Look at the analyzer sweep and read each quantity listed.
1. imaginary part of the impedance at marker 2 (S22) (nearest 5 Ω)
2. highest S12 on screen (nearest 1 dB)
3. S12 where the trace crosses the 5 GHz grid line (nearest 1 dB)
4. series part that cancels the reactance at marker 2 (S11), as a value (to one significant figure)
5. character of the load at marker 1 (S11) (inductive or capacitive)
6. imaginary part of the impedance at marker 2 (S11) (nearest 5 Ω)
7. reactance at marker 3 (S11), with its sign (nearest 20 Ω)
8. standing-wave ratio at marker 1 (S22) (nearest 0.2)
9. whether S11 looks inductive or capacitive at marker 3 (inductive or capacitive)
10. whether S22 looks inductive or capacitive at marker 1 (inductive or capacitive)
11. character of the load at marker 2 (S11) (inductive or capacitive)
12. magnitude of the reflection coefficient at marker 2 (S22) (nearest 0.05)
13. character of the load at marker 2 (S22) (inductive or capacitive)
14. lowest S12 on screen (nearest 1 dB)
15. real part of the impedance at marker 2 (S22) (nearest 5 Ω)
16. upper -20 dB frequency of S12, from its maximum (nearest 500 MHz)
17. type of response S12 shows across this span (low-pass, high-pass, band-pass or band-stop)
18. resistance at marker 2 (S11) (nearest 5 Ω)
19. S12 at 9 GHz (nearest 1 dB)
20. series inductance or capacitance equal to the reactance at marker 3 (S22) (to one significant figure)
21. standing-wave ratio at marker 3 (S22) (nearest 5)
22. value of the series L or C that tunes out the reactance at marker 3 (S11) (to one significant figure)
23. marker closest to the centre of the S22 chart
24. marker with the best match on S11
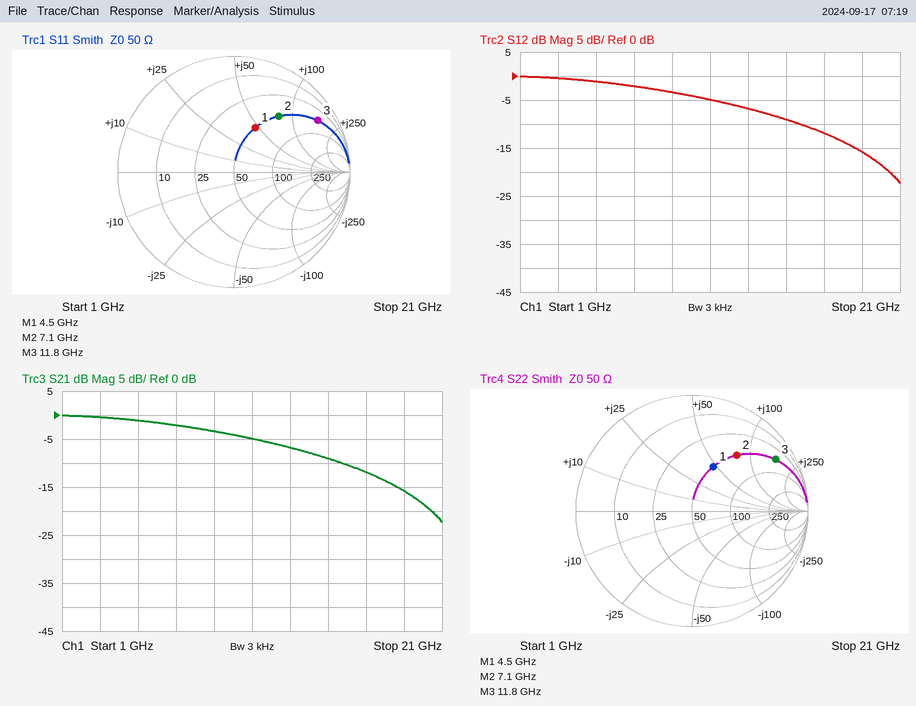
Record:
+80 Ω
0 dB
-1 dB
300 fF
inductive
+80 Ω
+160 Ω
2.4
inductive
inductive
inductive
0.60
inductive
-22 dB
50 Ω
20.5 GHz
low-pass
50 Ω
-3 dB
2 nH
10
80 fF
marker 1
marker 1
